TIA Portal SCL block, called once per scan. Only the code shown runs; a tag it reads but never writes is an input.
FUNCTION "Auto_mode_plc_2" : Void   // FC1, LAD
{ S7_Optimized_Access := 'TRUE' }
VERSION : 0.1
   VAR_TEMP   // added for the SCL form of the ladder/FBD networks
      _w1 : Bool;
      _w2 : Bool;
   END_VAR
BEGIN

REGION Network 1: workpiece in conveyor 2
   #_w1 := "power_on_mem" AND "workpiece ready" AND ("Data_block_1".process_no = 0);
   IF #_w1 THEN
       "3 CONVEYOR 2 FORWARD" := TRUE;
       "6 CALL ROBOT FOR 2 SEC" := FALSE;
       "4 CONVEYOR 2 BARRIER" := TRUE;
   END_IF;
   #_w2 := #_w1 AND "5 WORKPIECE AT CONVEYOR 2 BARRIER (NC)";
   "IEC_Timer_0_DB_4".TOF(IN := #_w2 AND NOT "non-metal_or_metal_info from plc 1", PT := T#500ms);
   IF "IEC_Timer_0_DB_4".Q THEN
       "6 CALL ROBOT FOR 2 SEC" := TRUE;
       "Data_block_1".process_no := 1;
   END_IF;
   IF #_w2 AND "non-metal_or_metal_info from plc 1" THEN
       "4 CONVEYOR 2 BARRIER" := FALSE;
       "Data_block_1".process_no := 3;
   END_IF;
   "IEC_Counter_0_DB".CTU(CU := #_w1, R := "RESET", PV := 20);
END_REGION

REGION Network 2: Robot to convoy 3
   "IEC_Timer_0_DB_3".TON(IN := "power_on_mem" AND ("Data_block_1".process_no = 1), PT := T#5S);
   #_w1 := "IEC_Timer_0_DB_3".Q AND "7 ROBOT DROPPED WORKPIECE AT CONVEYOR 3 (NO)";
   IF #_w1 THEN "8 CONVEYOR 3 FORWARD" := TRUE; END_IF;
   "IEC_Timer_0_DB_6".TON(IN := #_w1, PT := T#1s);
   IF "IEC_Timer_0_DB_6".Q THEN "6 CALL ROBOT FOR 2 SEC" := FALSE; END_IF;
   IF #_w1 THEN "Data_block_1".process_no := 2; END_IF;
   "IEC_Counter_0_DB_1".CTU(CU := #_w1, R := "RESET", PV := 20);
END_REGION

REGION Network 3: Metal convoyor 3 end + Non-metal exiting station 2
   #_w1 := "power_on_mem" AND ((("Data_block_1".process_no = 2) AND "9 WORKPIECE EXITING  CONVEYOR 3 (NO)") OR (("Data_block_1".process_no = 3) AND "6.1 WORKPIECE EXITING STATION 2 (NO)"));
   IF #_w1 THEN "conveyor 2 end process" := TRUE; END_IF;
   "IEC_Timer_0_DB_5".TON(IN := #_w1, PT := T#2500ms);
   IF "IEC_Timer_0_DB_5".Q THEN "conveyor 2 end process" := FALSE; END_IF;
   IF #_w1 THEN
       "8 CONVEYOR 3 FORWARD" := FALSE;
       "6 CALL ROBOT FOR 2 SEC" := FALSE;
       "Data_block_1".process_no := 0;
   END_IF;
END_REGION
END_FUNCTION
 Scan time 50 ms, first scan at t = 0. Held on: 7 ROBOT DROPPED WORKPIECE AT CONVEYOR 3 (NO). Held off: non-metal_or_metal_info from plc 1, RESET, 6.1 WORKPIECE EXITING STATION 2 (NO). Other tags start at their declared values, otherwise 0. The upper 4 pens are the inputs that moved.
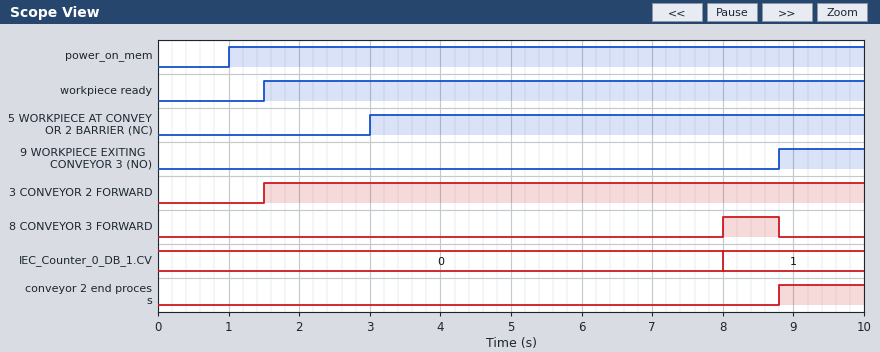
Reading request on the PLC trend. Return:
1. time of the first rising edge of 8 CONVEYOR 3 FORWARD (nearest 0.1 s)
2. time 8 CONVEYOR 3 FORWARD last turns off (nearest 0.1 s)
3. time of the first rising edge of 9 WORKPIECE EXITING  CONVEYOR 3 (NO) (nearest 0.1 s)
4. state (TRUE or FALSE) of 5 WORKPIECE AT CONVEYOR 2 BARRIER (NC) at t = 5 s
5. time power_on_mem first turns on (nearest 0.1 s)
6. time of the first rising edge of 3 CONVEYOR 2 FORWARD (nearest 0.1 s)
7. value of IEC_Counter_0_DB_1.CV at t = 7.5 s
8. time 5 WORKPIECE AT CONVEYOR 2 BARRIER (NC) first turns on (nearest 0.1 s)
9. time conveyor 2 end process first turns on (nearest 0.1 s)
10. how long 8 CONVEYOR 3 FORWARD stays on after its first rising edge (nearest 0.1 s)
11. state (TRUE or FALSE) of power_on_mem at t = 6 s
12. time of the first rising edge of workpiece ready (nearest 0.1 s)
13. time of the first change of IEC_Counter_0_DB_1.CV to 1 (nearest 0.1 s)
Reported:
8.0 s
8.8 s
8.8 s
TRUE
1.0 s
1.5 s
0
3.0 s
8.8 s
0.8 s
TRUE
1.5 s
8.0 s
